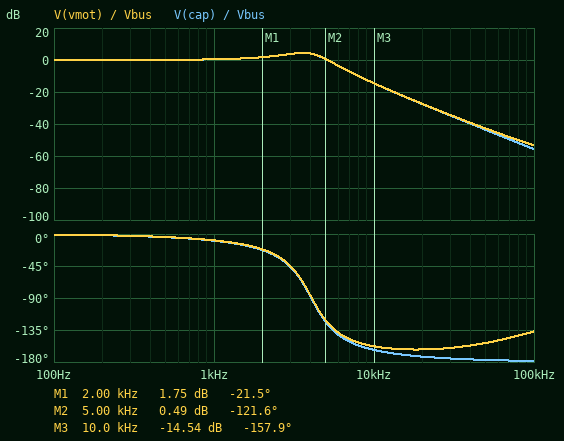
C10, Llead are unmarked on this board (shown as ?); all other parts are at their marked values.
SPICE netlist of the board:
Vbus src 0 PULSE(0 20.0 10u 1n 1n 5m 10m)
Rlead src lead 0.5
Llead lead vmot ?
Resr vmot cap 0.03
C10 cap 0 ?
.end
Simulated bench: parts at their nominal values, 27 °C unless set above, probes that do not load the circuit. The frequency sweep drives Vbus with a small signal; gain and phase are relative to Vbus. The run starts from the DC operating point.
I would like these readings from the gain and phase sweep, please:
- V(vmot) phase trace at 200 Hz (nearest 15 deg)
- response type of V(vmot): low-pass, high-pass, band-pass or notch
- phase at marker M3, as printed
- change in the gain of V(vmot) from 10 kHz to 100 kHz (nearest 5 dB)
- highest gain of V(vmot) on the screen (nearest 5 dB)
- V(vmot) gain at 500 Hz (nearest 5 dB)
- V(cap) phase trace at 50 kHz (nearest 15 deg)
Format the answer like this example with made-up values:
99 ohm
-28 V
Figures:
0 deg
low-pass
-157.9 deg
-40 dB
5 dB
0 dB
-180 deg
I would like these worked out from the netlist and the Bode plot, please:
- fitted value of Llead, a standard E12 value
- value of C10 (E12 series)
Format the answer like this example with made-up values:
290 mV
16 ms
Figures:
33 µH
47 µF
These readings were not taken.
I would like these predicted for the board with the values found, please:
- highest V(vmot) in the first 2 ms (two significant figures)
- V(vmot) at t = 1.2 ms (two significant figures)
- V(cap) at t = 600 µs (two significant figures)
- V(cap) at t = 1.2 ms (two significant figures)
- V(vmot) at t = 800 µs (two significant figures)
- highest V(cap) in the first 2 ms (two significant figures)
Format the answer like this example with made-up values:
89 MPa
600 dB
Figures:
27 V
20 V
20 V
20 V
20 V
27 V
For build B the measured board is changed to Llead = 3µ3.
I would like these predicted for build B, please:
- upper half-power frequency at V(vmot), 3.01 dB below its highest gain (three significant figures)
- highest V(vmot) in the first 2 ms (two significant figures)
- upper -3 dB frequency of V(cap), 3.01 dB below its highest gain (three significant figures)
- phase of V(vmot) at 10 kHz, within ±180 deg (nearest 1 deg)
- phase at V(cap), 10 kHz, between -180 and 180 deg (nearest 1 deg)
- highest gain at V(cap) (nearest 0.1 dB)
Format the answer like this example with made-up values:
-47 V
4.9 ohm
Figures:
8.26 kHz
20 V
8.22 kHz
-71 deg
-76 deg
0 dB
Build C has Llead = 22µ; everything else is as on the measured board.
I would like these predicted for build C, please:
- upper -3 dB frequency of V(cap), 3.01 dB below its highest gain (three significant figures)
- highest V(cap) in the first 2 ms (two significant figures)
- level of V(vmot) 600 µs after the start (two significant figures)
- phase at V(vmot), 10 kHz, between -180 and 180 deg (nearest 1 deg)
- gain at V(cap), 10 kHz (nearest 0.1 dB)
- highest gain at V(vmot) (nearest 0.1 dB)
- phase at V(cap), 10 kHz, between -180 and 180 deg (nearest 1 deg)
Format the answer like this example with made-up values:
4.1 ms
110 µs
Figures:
5.89 kHz
25 V
20 V
-148 deg
-10.8 dB
2.9 dB
-153 deg
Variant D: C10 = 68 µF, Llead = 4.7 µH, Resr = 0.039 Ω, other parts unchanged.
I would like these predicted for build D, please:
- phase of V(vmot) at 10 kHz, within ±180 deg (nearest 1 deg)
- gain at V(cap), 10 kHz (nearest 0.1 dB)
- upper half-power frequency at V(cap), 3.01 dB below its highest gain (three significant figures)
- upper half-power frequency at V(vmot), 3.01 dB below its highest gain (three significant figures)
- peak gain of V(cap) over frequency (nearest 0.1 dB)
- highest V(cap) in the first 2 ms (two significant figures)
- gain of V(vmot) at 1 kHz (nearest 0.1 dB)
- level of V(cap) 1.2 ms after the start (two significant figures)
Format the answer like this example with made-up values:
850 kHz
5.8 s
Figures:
-87 deg
-7.3 dB
5.53 kHz
5.57 kHz
0 dB
20 V
-0.1 dB
20 V
